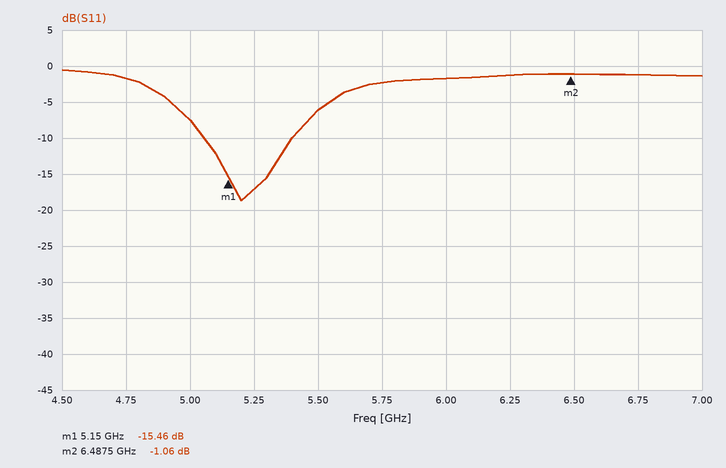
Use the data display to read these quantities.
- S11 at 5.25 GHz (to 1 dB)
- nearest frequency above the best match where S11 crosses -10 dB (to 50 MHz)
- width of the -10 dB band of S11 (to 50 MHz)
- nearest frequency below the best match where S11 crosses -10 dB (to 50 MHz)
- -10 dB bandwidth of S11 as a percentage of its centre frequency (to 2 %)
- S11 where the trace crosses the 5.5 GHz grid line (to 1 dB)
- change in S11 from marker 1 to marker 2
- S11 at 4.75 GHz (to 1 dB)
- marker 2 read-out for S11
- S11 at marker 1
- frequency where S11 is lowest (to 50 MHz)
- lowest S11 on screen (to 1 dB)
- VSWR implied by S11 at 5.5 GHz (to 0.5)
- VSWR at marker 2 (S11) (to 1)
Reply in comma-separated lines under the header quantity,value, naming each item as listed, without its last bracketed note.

quantity,value
S11 at 5.25 GHz,-17 dB
nearest frequency above the best match where S11 crosses -10 dB,5.40 GHz
width of the -10 dB band of S11,350 MHz
nearest frequency below the best match where S11 crosses -10 dB,5.05 GHz
-10 dB bandwidth of S11 as a percentage of its centre frequency,6 %
S11 where the trace crosses the 5.5 GHz grid line,-6 dB
change in S11 from marker 1 to marker 2,14.40 dB
S11 at 4.75 GHz,-2 dB
marker 2 read-out for S11,-1.06 dB
S11 at marker 1,-15.46 dB
frequency where S11 is lowest,5.20 GHz
lowest S11 on screen,-19 dB
VSWR implied by S11 at 5.5 GHz,3.0
VSWR at marker 2 (S11),16
